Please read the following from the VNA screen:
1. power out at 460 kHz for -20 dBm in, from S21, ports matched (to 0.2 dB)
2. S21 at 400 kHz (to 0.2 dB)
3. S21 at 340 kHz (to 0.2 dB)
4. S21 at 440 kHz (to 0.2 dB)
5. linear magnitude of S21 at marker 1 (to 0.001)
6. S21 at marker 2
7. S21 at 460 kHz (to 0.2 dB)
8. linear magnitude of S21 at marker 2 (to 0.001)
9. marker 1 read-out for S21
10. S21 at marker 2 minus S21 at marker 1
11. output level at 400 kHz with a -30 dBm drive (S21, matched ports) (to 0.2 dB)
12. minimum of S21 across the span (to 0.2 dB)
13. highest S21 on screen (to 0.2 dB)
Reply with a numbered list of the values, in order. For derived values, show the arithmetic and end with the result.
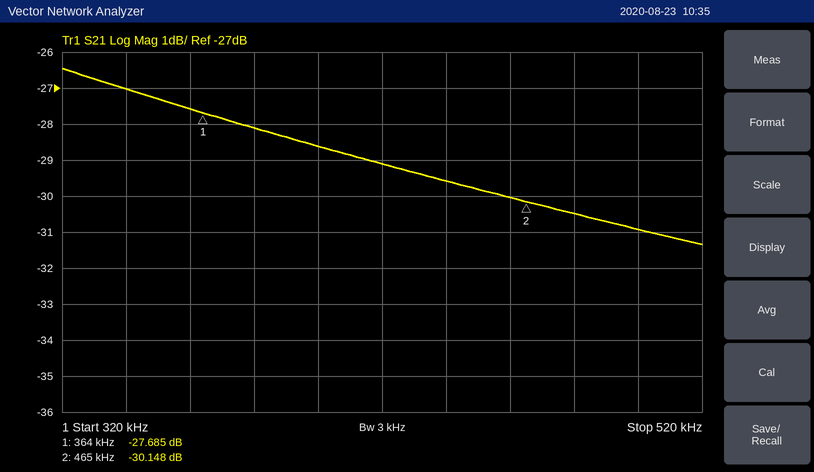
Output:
1. -20 dBm + (-30.0 dB) = -50.0 dBm
2. -28.6 dB
3. -27.0 dB
4. -29.6 dB
5. 10^(-27.685/20) ≈ 0.041
6. -30.148 dB
7. -30.0 dB
8. 10^(-30.148/20) ≈ 0.031
9. -27.685 dB
10. -30.148 − (-27.685) = -2.463 dB
11. -30 dBm + (-28.6 dB) = -58.6 dBm
12. -31.4 dB
13. -26.4 dB
